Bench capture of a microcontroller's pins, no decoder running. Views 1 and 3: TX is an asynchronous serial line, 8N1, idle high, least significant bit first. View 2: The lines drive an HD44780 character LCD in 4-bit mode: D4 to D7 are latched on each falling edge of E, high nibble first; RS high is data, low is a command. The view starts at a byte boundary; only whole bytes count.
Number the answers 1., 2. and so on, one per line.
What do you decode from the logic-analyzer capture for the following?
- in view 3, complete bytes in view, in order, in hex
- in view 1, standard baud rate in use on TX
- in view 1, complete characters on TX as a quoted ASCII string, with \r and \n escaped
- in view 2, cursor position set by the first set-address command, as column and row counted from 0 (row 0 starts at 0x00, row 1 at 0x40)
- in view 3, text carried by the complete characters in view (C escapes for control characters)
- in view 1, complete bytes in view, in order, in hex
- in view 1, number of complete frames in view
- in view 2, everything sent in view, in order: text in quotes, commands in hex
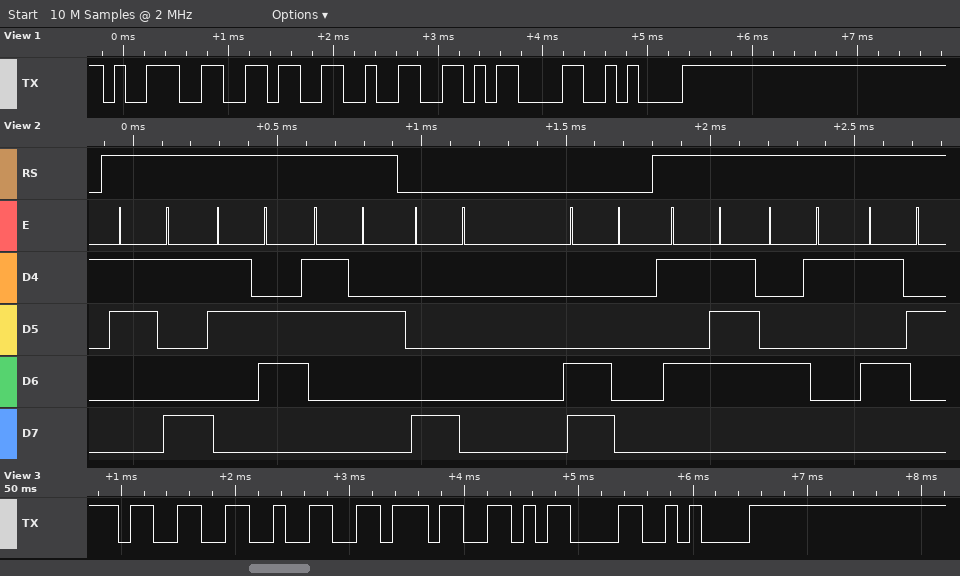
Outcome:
1. 33 32 37 0D 0A
2. 9600 baud
3. "962\r\n"
4. column 0, row 0
5. "327\r\n"
6. 39 36 32 0D 0A
7. 5
8. "962" 0x80 0xC0 "WAR"
